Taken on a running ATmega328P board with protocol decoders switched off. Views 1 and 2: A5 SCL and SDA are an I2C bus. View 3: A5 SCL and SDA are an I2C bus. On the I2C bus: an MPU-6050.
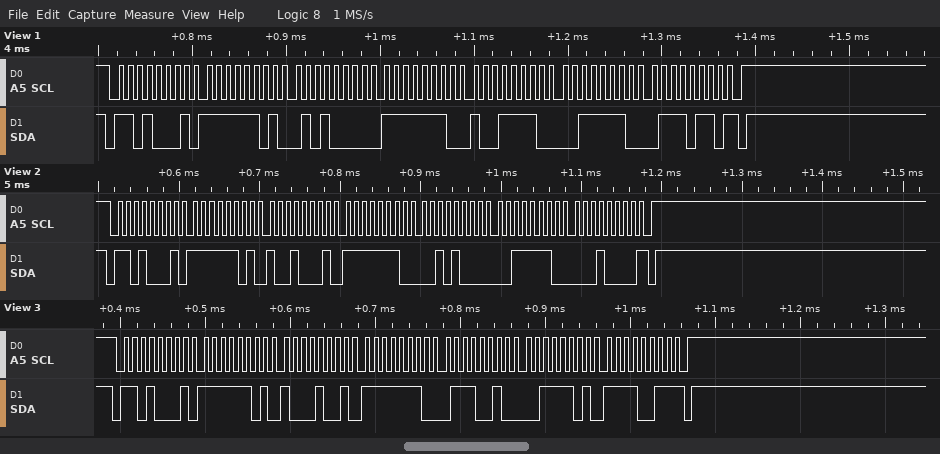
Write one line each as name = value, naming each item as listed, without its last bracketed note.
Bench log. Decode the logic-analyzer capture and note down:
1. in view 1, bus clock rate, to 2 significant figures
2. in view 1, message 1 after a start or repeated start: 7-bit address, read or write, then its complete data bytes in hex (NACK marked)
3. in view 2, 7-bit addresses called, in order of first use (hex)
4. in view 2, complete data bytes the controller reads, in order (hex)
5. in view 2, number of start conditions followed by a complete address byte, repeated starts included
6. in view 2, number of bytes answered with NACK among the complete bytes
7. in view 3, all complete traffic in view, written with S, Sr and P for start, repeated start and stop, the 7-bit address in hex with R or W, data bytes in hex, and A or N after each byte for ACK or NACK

in view 1, bus clock rate, to 2 significant figures = 100 kHz
in view 1, message 1 after a start or repeated start: 7-bit address, read or write, then its complete data bytes in hex = 0x68 read: FD 50 FE 9E 3E 76 NACK
in view 2, 7-bit addresses called, in order of first use = 0x68
in view 2, complete data bytes the controller reads, in order = FD 91 FE 28 3E 10
in view 2, number of start conditions followed by a complete address byte, repeated starts included = 1
in view 2, number of bytes answered with NACK among the complete bytes = 1
in view 3, all complete traffic in view, written with S, Sr and P for start, repeated start and stop, the 7-bit address in hex with R or W, data bytes in hex, and A or N after each byte for ACK or NACK = S 68R A FD A 89 A FE A 72 A 3D A F3 N P
